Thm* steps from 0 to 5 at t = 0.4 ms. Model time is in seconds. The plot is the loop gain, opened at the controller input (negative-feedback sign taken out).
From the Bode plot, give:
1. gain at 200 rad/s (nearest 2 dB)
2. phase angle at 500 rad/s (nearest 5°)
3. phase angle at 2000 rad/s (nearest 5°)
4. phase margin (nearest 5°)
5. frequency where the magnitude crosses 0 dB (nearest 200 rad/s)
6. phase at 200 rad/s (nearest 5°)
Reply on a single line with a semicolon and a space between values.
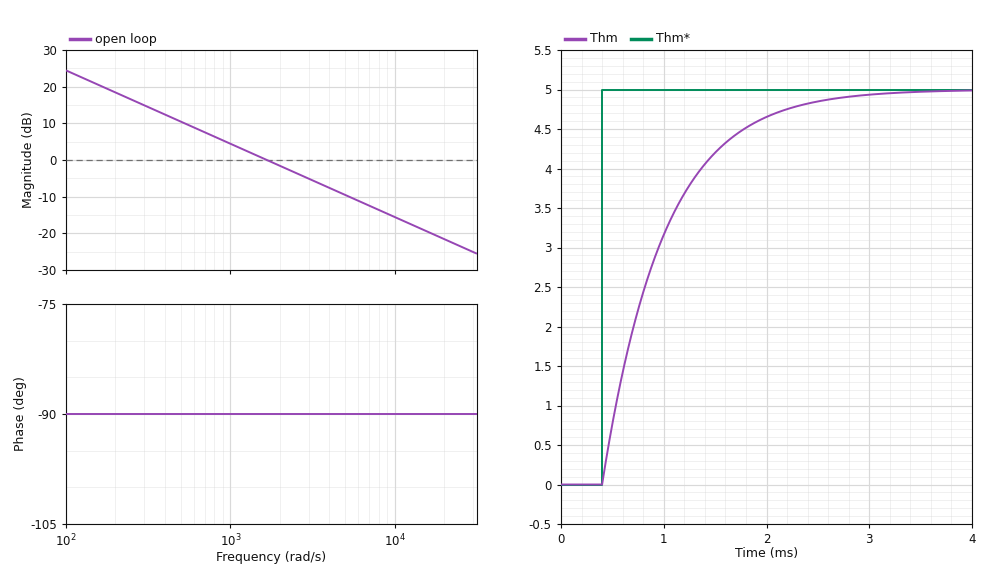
18 dB; -90°; -90°; 90°; 1600 rad/s; -90°
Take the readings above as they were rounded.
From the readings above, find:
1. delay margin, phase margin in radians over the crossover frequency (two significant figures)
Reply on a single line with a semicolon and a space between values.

0.00098 s
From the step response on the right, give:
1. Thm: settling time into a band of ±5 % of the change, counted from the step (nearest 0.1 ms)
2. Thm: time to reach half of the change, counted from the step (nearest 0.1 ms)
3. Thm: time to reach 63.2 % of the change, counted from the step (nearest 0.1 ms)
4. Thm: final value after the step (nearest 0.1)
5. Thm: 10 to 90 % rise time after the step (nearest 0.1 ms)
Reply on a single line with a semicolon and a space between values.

1.8 ms; 0.4 ms; 0.6 ms; 5.0; 1.3 ms
